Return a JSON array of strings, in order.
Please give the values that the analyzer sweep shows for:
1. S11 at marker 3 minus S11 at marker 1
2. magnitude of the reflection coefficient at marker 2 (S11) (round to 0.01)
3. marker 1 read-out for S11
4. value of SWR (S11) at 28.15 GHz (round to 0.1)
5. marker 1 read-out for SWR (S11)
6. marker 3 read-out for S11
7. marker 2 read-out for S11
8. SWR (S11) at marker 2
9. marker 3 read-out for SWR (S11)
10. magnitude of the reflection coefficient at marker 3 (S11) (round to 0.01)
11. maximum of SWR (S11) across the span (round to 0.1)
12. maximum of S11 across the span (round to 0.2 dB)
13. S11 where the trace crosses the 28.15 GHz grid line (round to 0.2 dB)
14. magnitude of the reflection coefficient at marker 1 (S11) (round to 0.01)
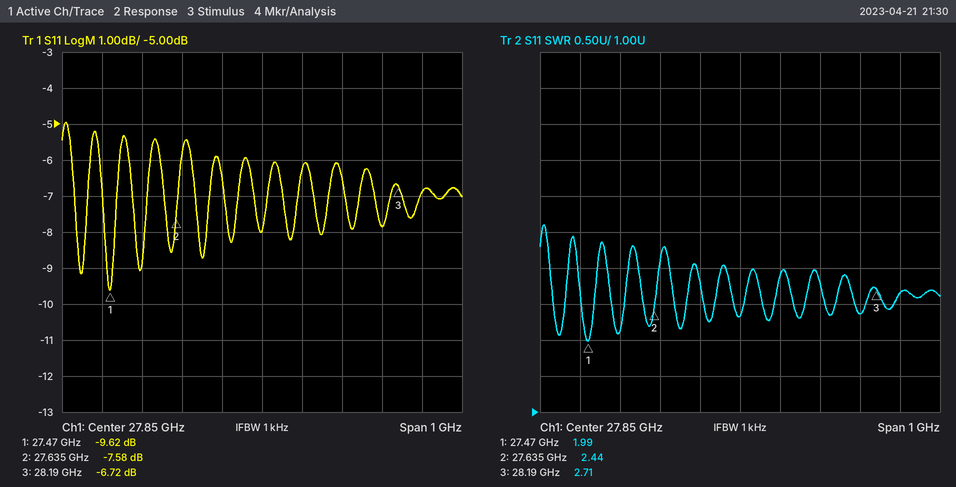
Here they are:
["2.90 dB", "0.42", "-9.62 dB", "2.4", "1.99", "-6.72 dB", "-7.58 dB", "2.44", "2.71", "0.46", "3.6", "-5.0 dB", "-7.8 dB", "0.33"]
